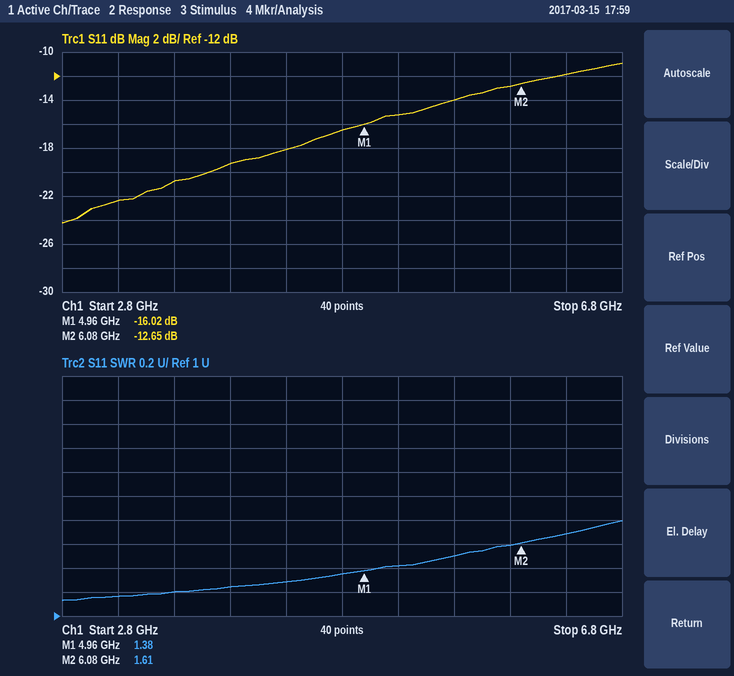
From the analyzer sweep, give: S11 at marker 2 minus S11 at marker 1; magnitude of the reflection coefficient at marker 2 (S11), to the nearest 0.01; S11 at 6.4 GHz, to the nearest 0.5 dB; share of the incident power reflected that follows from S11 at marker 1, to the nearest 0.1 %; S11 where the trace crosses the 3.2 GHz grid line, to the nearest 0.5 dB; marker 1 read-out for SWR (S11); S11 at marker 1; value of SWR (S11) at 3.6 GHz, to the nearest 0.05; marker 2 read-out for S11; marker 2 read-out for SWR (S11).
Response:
3.37 dB
0.23
-12.0 dB
2.5 %
-22.5 dB
1.38
-16.02 dB
1.20
-12.65 dB
1.61
